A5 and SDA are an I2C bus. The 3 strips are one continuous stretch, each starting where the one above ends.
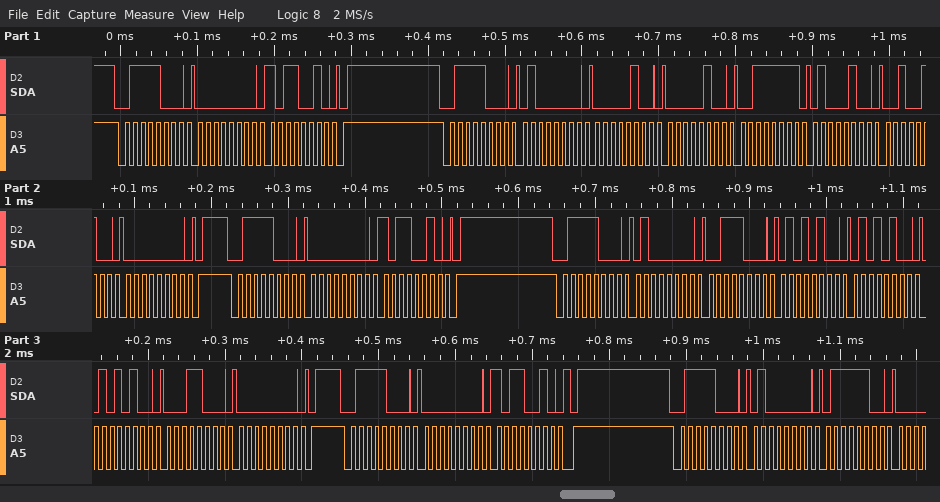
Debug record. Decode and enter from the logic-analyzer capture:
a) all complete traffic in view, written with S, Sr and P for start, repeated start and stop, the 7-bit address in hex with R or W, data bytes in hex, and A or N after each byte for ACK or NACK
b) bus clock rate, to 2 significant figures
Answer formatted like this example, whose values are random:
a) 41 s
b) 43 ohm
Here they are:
a) S 3CW A 00 A B2 A P S 3CW A 40 A 04 A 04 A 3F A 44 A 24 A 00 A P S 3CW A 00 A B2 A P S 3CW A 40 A 38 A 54 A 54 A 54 A 18 A 00 A P S 3CW A 00 A B2 A P S 3CW A 40 A 7C A
b) 100 kHz
